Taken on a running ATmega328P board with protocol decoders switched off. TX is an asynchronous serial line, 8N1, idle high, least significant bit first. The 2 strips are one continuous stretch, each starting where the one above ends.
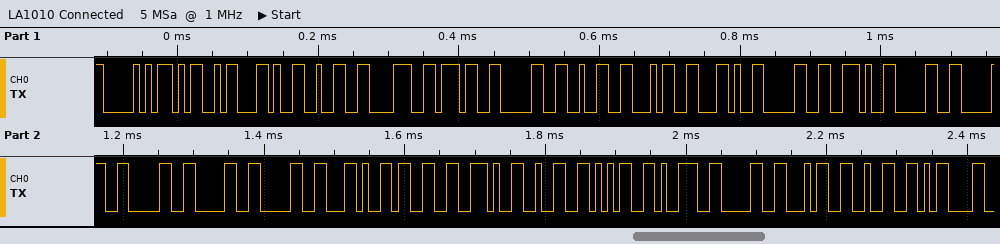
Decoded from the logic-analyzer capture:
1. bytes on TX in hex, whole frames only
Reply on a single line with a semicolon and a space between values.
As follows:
0x50 0x4D 0x2C 0x32 0x38 0x37 0x30 0x32 0x34 0x2C 0x30 0x2E 0x30 0x30 0x30 0x30 0x30 0x2C 0x33 0x2E 0x32 0x35 0x39 0x30 0x34 0x32 0x0D
